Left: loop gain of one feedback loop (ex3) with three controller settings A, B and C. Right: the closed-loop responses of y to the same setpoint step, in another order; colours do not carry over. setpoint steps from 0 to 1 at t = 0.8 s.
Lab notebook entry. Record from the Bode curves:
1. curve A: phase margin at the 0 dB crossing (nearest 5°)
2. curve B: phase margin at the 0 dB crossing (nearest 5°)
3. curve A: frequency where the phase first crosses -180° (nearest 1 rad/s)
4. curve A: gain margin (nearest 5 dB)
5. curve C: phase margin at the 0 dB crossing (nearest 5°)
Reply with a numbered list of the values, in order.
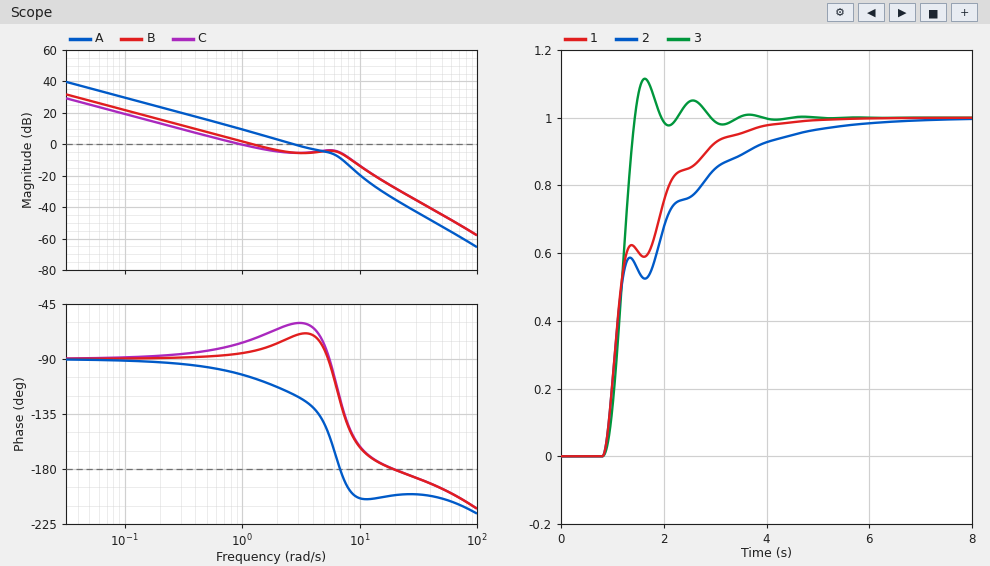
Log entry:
1. 60°
2. 95°
3. 7 rad/s
4. 10 dB
5. 105°
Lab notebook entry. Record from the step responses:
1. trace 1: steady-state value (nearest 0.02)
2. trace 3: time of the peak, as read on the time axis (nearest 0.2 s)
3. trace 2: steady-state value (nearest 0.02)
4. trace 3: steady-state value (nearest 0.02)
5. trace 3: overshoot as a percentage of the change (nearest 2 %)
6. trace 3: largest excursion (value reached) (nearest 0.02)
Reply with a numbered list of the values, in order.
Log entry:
1. 1.00
2. 1.6 s
3. 1.00
4. 1.00
5. 12 %
6. 1.12
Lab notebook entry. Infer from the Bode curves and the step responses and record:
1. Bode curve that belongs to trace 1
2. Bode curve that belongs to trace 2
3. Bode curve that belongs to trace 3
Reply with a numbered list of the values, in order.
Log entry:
1. B
2. C
3. A
